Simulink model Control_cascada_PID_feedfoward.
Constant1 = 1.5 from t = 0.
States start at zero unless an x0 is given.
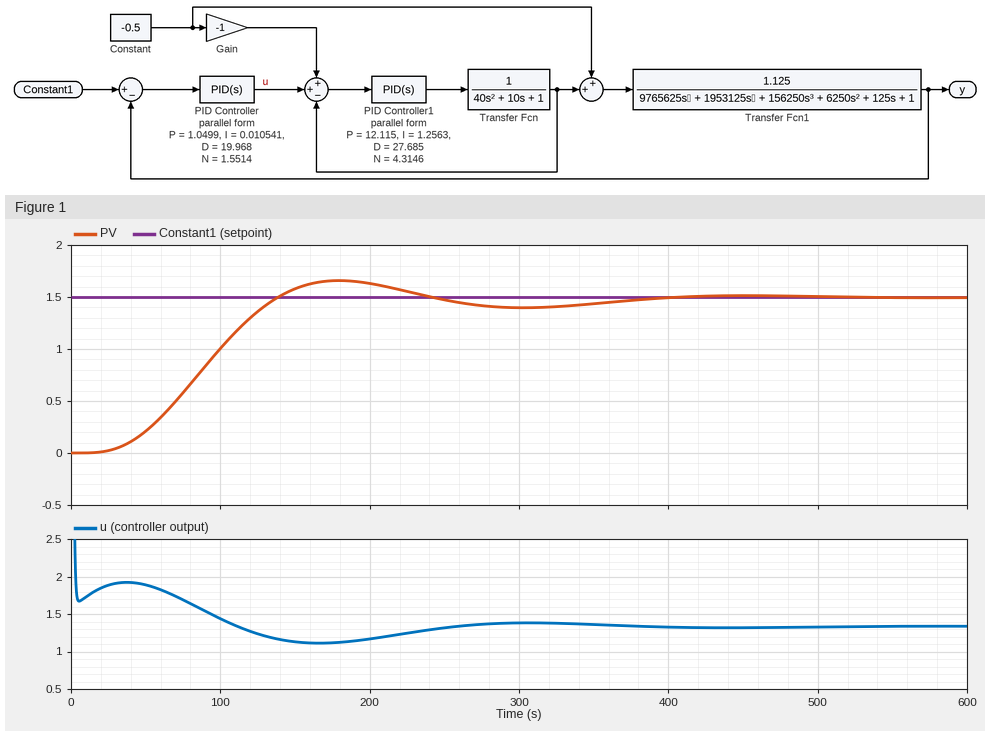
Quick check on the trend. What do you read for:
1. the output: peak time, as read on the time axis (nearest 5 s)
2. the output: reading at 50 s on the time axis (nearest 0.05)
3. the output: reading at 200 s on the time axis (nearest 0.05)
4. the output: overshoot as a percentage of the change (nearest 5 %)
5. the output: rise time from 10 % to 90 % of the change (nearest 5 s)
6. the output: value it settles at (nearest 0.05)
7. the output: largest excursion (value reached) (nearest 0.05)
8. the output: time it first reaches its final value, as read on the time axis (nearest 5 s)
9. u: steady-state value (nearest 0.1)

180 s
0.20
1.65
10 %
80 s
1.50
1.65
140 s
1.3
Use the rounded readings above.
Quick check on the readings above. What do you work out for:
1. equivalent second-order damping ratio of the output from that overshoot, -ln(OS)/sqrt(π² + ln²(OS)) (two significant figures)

0.59
